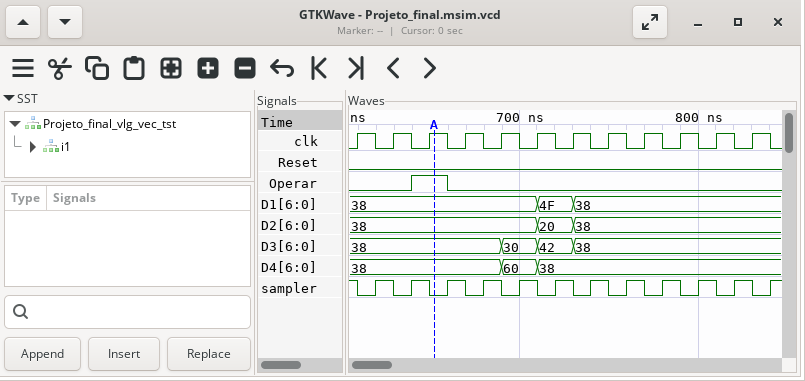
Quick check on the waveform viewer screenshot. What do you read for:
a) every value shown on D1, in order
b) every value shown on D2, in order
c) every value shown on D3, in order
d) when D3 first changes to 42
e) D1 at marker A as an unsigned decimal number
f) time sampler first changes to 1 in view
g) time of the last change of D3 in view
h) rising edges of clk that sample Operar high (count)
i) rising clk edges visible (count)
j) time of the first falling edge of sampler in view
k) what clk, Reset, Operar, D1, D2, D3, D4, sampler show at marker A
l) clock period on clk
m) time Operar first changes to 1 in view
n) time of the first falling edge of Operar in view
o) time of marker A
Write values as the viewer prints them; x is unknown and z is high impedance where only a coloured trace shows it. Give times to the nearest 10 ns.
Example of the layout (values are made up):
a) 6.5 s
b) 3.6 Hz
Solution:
a) 38, 4F, 38
b) 38, 20, 38
c) 38, 30, 42, 38
d) 710 ns
e) 56
f) 620 ns
g) 730 ns
h) 1
i) 12
j) 610 ns
k) clk=1, Reset=0, Operar=1, D1=38, D2=38, D3=38, D4=38, sampler=0
l) 20 ns
m) 640 ns
n) 660 ns
o) 650 ns
